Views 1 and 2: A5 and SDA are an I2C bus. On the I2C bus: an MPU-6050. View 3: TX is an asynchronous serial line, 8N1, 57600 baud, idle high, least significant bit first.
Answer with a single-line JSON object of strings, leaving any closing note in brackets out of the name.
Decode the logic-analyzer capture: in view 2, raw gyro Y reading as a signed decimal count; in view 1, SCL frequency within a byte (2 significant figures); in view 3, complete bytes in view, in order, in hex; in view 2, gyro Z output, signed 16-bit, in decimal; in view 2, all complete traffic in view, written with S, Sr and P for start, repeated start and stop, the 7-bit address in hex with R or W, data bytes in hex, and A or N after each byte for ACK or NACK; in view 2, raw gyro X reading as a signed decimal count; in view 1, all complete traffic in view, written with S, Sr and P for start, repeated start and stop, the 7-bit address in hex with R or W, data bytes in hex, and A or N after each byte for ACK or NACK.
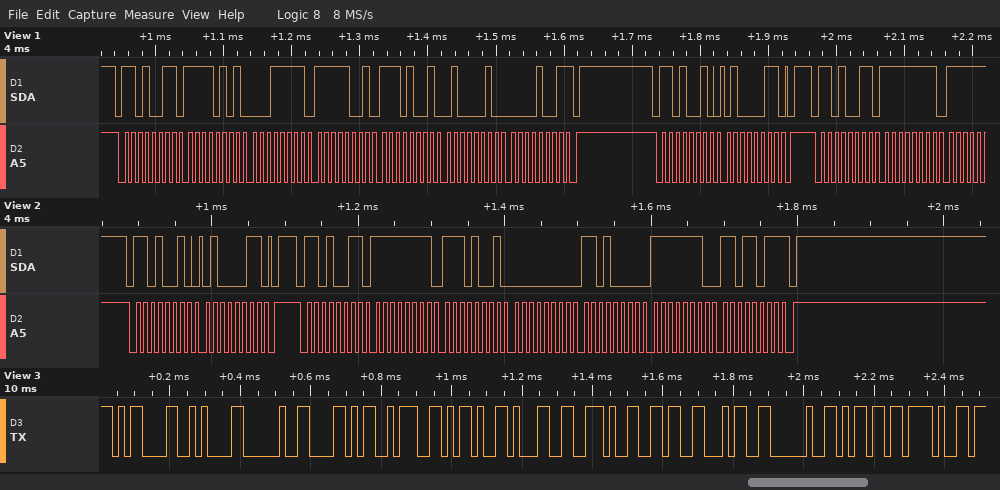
{"in view 2, raw gyro Y reading as a signed decimal count": "208", "in view 1, SCL frequency within a byte": "100 kHz", "in view 3, complete bytes in view, in order, in hex": "0x0D 0x0A 0x20 0x58 0x3A 0x2D 0x31 0x2E 0x36 0x34 0x20 0x6D 0x2F", "in view 2, gyro Z output, signed 16-bit, in decimal": "-293", "in view 2, all complete traffic in view, written with S, Sr and P for start, repeated start and stop, the 7-bit address in hex with R or W, data bytes in hex, and A or N after each byte for ACK or NACK": "S 69W A 43 A P S 69R A FF A E9 A 00 A D0 A FE A DB N P", "in view 2, raw gyro X reading as a signed decimal count": "-23", "in view 1, all complete traffic in view, written with S, Sr and P for start, repeated start and stop, the 7-bit address in hex with R or W, data bytes in hex, and A or N after each byte for ACK or NACK": "S 69R A F5 A 1F A F9 A E9 A 42 A 09 N P S 69W A 43 A P S 69R A FF A"}
